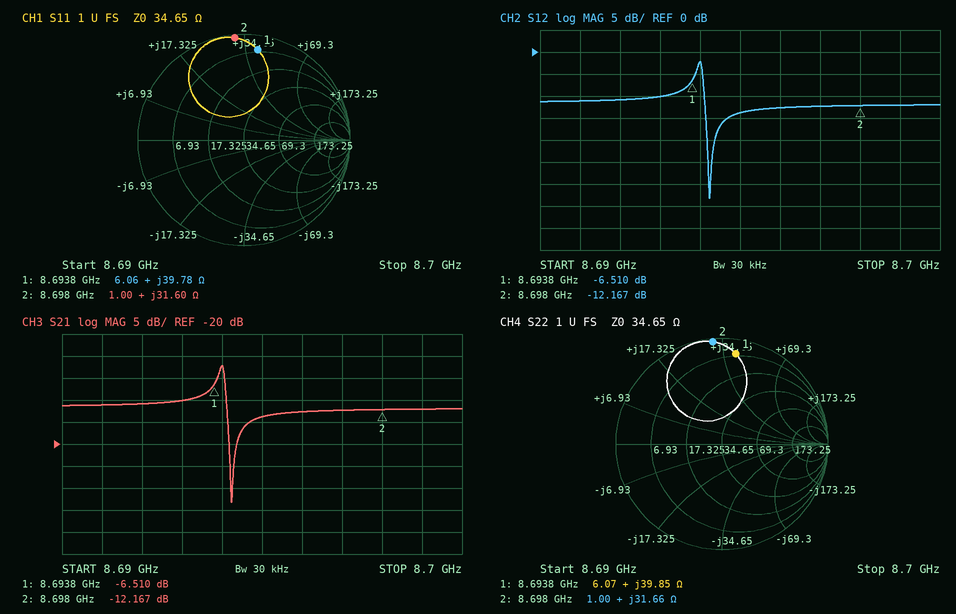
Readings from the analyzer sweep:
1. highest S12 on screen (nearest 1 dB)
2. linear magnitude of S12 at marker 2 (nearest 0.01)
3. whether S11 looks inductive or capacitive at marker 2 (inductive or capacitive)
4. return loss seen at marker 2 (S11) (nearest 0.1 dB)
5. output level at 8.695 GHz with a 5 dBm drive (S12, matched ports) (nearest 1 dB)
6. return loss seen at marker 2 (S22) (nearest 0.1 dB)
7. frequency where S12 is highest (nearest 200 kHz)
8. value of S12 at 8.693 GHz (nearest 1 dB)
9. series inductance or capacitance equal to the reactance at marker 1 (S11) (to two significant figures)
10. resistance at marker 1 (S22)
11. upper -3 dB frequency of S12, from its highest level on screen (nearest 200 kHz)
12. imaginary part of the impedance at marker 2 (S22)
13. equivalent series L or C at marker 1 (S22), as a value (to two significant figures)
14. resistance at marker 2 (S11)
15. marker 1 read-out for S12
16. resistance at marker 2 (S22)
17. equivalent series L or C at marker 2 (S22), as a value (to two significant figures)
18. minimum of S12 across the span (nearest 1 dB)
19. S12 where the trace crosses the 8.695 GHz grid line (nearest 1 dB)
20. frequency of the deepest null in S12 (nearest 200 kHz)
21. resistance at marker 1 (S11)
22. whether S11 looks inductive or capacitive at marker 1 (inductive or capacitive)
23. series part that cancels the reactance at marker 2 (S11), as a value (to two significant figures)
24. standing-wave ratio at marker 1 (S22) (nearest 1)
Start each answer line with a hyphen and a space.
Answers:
- -2 dB
- 0.25
- inductive
- 0.3 dB
- -9 dBm
- 0.3 dB
- 8.6940 GHz
- -10 dB
- 730 pH
- 6.07 Ω
- 8.6940 GHz
- +31.66 Ω
- 730 pH
- 1.00 Ω
- -6.510 dB
- 1.00 Ω
- 580 pH
- -33 dB
- -14 dB
- 8.6942 GHz
- 6.06 Ω
- inductive
- 580 fF
- 13
